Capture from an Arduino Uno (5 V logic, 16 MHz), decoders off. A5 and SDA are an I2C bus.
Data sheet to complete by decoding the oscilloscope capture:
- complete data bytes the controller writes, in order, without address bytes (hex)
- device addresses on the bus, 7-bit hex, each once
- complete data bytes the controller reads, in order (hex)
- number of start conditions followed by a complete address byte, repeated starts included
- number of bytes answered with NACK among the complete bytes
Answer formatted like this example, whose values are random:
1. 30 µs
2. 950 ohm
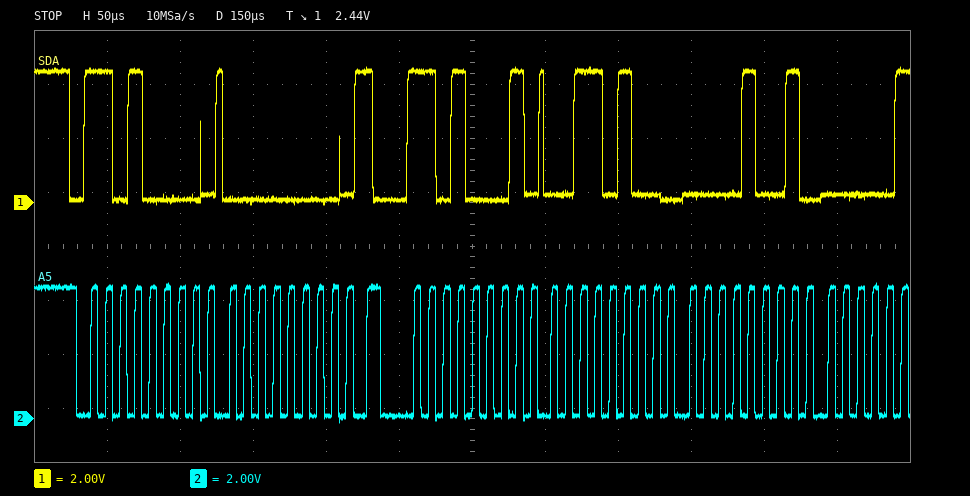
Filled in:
1. 00
2. 0x68
3. 34 09
4. 2
5. 0
